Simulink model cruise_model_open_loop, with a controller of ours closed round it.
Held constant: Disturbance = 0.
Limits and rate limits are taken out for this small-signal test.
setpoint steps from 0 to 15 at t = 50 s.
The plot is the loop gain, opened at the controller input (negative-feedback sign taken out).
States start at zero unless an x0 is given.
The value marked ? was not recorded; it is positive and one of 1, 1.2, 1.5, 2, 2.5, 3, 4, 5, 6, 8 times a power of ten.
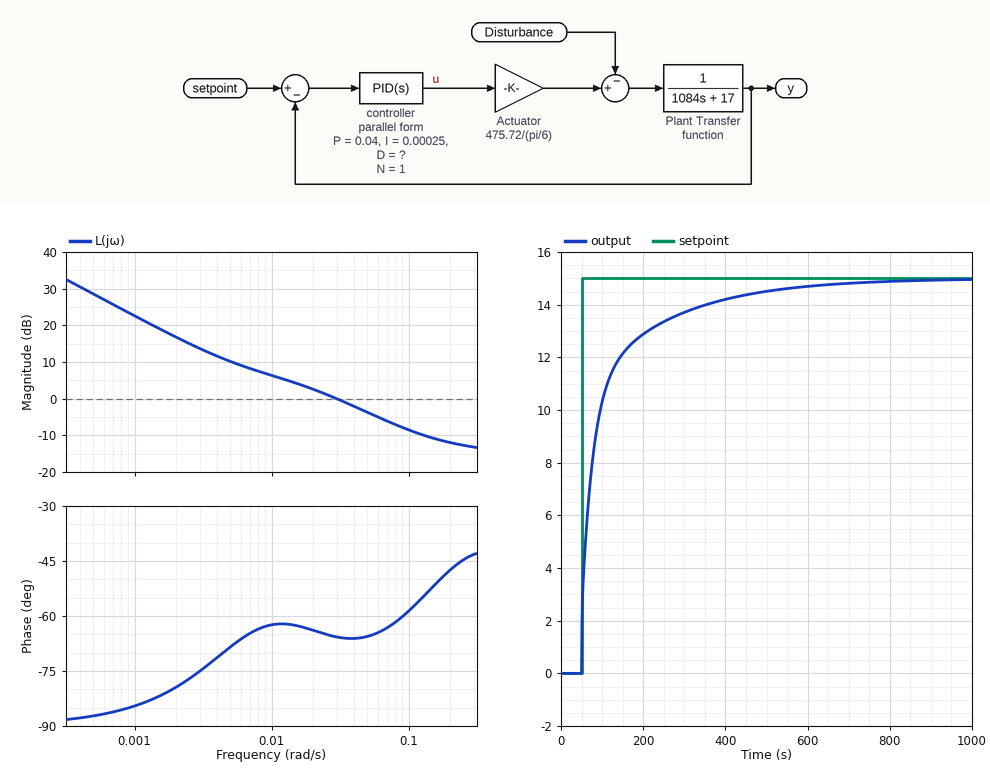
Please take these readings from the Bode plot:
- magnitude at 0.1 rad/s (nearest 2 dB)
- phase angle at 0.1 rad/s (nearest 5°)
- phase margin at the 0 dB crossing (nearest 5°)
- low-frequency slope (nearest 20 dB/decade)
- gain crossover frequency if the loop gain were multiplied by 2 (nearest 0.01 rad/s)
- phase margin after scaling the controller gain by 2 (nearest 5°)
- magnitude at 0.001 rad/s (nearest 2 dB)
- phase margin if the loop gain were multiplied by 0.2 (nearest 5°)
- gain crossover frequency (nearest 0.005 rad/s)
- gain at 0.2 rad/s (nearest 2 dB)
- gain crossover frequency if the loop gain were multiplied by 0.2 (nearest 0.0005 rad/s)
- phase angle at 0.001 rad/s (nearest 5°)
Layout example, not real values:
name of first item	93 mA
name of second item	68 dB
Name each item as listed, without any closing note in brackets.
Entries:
magnitude at 0.1 rad/s	-8 dB
phase angle at 0.1 rad/s	-60°
phase margin at the 0 dB crossing	115°
low-frequency slope	-20 dB/decade
gain crossover frequency if the loop gain were multiplied by 2	0.07 rad/s
phase margin after scaling the controller gain by 2	115°
magnitude at 0.001 rad/s	22 dB
phase margin if the loop gain were multiplied by 0.2	105°
gain crossover frequency	0.030 rad/s
gain at 0.2 rad/s	-12 dB
gain crossover frequency if the loop gain were multiplied by 0.2	0.0030 rad/s
phase angle at 0.001 rad/s	-85°
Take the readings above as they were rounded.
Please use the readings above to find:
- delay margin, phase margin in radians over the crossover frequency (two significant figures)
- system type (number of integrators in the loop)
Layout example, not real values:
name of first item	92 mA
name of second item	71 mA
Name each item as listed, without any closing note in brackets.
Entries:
delay margin, phase margin in radians over the crossover frequency	67 s
system type	1
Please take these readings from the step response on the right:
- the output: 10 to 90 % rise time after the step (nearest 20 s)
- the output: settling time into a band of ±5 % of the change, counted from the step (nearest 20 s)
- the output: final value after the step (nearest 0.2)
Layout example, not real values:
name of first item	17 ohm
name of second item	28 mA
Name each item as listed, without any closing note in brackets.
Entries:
the output: 10 to 90 % rise time after the step	220 s
the output: settling time into a band of ±5 % of the change, counted from the step	360 s
the output: final value after the step	15.0
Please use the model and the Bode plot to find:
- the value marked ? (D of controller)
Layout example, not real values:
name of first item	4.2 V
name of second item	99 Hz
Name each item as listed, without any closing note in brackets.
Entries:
the value marked ?	0.2
